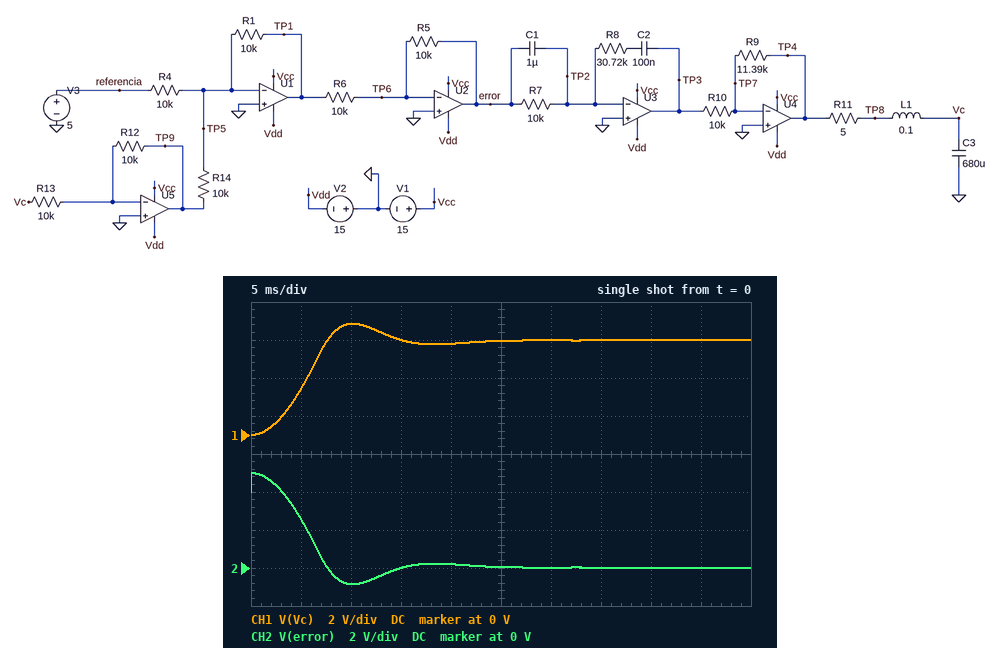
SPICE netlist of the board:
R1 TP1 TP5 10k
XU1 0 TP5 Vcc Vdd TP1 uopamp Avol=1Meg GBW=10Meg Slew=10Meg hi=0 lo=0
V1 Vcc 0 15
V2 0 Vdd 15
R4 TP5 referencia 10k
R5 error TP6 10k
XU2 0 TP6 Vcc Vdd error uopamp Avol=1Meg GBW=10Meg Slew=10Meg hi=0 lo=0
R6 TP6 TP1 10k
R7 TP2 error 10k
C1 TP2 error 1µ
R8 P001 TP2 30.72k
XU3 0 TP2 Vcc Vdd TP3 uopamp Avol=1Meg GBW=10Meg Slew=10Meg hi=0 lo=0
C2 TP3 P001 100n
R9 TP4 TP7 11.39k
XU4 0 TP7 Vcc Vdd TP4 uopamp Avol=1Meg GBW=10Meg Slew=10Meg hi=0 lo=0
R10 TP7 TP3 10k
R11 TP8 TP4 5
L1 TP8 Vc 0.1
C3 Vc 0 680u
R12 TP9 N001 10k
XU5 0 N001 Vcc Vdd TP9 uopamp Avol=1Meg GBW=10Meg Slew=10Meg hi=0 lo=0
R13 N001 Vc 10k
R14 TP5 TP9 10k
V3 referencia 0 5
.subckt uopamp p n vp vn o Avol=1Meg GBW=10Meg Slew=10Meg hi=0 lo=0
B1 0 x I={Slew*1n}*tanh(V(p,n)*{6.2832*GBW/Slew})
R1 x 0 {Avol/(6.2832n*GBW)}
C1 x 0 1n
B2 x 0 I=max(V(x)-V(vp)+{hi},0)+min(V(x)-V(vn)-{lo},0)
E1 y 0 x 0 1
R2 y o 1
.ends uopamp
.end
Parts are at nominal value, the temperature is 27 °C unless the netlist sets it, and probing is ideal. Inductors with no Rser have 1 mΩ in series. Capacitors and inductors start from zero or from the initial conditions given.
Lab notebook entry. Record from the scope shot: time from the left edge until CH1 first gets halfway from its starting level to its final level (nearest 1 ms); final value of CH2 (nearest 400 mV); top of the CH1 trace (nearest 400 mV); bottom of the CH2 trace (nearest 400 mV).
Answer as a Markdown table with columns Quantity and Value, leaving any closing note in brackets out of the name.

| Quantity | Value |
|---|---|
| time from the left edge until CH1 first gets halfway from its starting level to its final level | 5 ms |
| final value of CH2 | 0 V |
| top of the CH1 trace | 6.0 V |
| bottom of the CH2 trace | -800 mV |
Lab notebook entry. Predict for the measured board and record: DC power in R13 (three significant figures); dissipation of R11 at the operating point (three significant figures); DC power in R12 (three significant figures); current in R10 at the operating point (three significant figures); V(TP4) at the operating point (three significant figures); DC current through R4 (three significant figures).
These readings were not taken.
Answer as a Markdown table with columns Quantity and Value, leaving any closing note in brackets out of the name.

| Quantity | Value |
|---|---|
| DC power in R13 | 2.50 mW |
| dissipation of R11 at the operating point | 1.25 µW |
| DC power in R12 | 2.50 mW |
| current in R10 at the operating point | 439 µA |
| V(TP4) at the operating point | 5.00 V |
| DC current through R4 | 500 µA |
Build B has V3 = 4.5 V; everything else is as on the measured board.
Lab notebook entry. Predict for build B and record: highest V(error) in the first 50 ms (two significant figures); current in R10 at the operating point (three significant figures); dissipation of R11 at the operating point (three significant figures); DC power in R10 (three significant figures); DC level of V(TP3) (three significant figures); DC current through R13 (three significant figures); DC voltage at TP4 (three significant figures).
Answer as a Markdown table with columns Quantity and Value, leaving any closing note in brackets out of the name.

| Quantity | Value |
|---|---|
| highest V(error) in the first 50 ms | 4.5 V |
| current in R10 at the operating point | 395 µA |
| dissipation of R11 at the operating point | 1.01 µW |
| DC power in R10 | 1.56 mW |
| DC level of V(TP3) | -3.95 V |
| DC current through R13 | 450 µA |
| DC voltage at TP4 | 4.50 V |
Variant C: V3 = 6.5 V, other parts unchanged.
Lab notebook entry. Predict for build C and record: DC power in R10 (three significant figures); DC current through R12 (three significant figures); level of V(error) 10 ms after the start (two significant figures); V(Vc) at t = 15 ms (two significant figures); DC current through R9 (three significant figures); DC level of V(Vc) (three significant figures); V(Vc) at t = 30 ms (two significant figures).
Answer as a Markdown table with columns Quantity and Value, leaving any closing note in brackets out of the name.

| Quantity | Value |
|---|---|
| DC power in R10 | 3.26 mW |
| DC current through R12 | 650 µA |
| level of V(error) 10 ms after the start | -790 mV |
| V(Vc) at t = 15 ms | 6.8 V |
| DC current through R9 | 571 µA |
| DC level of V(Vc) | 6.50 V |
| V(Vc) at t = 30 ms | 6.5 V |
